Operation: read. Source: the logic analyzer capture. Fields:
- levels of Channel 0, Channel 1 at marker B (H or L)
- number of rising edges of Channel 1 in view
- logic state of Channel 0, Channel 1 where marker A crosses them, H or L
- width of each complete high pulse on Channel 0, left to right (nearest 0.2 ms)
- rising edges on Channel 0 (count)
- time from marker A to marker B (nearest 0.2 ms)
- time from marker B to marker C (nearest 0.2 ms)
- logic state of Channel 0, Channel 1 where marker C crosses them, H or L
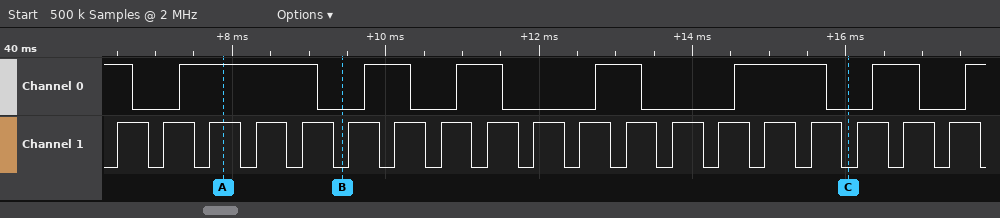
Channel 0=L, Channel 1=L
19
Channel 0=H, Channel 1=H
1.8 ms, 0.6 ms, 0.6 ms, 0.6 ms, 1.2 ms, 0.6 ms
7
1.6 ms
6.6 ms
Channel 0=L, Channel 1=L
